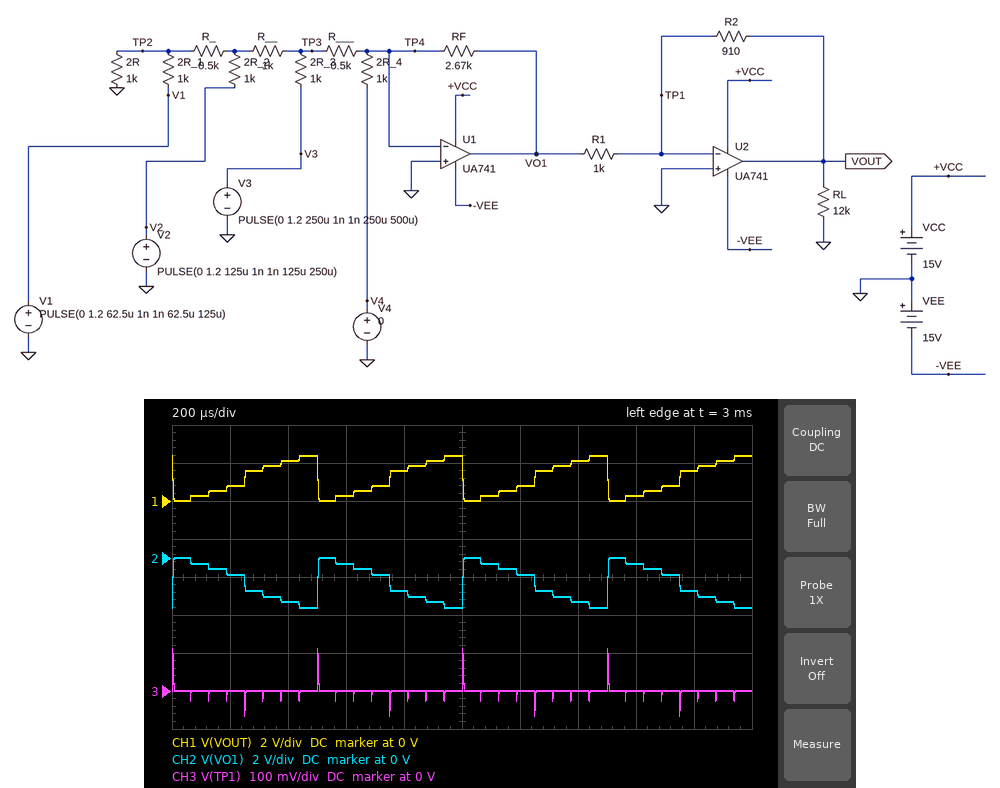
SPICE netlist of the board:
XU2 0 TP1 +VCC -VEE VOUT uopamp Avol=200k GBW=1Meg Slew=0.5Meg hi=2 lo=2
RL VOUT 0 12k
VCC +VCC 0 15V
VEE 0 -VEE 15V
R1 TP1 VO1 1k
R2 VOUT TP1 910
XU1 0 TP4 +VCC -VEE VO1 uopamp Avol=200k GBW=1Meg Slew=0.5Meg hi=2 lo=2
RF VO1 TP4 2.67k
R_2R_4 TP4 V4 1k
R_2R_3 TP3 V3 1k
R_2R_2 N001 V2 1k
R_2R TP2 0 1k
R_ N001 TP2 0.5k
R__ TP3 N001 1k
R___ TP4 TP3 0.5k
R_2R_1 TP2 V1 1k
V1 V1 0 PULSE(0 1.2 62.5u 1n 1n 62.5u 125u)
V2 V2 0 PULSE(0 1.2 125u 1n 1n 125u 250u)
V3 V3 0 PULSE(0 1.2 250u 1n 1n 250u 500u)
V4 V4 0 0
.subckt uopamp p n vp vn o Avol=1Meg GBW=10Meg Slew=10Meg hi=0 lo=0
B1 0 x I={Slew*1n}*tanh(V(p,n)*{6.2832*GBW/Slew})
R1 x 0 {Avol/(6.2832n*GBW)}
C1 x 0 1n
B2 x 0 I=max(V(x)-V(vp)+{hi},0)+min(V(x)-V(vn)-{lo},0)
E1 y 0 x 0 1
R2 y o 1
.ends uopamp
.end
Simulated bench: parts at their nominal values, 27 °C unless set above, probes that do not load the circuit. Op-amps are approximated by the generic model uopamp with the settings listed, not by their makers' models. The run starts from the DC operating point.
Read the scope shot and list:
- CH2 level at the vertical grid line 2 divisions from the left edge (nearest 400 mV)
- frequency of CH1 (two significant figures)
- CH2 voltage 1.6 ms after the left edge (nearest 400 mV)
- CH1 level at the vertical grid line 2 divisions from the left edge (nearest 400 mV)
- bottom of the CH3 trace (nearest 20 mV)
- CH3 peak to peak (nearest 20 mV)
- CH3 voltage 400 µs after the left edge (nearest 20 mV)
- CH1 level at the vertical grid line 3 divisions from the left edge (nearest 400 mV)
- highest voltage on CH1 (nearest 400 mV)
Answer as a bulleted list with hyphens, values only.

- -2.4 V
- 2.0 kHz
- -400 mV
- 2.0 V
- -60 mV
- 180 mV
- 0 V
- 400 mV
- 2.4 V
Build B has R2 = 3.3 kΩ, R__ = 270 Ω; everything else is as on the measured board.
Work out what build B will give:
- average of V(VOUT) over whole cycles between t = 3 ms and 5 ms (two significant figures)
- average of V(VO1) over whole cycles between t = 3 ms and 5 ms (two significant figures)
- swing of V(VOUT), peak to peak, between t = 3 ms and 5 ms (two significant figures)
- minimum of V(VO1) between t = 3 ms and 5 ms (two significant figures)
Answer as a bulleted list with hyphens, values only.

- 5.0 V
- -1.5 V
- 9.7 V
- -2.9 V
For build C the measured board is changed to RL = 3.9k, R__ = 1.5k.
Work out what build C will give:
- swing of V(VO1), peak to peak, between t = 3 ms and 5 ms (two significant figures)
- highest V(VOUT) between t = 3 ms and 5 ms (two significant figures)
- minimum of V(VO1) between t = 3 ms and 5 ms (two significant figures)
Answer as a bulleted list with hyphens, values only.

- 2.5 V
- 2.3 V
- -2.5 V
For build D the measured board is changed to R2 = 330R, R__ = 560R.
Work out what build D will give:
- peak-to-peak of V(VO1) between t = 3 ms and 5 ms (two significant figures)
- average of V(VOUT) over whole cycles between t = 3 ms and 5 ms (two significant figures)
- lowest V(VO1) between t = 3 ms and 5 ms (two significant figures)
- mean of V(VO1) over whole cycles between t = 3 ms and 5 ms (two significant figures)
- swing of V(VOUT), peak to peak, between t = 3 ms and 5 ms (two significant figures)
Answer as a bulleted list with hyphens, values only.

- 2.8 V
- 460 mV
- -2.8 V
- -1.4 V
- 920 mV
